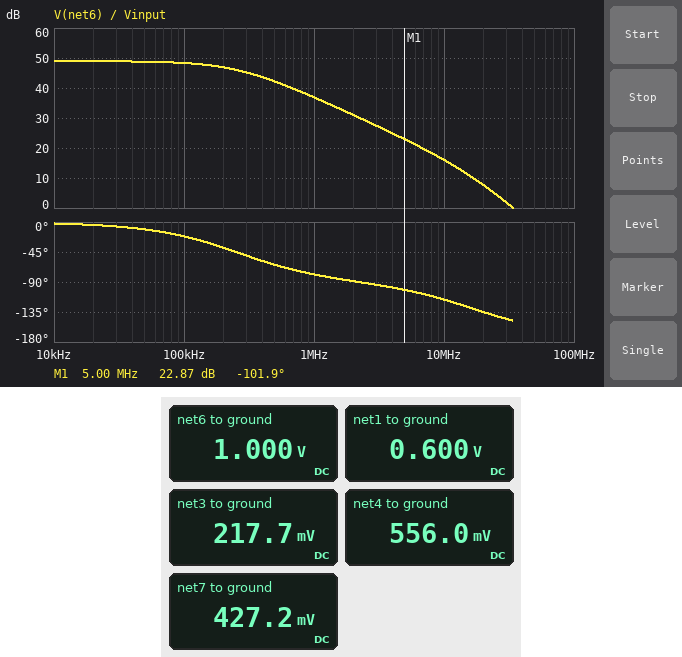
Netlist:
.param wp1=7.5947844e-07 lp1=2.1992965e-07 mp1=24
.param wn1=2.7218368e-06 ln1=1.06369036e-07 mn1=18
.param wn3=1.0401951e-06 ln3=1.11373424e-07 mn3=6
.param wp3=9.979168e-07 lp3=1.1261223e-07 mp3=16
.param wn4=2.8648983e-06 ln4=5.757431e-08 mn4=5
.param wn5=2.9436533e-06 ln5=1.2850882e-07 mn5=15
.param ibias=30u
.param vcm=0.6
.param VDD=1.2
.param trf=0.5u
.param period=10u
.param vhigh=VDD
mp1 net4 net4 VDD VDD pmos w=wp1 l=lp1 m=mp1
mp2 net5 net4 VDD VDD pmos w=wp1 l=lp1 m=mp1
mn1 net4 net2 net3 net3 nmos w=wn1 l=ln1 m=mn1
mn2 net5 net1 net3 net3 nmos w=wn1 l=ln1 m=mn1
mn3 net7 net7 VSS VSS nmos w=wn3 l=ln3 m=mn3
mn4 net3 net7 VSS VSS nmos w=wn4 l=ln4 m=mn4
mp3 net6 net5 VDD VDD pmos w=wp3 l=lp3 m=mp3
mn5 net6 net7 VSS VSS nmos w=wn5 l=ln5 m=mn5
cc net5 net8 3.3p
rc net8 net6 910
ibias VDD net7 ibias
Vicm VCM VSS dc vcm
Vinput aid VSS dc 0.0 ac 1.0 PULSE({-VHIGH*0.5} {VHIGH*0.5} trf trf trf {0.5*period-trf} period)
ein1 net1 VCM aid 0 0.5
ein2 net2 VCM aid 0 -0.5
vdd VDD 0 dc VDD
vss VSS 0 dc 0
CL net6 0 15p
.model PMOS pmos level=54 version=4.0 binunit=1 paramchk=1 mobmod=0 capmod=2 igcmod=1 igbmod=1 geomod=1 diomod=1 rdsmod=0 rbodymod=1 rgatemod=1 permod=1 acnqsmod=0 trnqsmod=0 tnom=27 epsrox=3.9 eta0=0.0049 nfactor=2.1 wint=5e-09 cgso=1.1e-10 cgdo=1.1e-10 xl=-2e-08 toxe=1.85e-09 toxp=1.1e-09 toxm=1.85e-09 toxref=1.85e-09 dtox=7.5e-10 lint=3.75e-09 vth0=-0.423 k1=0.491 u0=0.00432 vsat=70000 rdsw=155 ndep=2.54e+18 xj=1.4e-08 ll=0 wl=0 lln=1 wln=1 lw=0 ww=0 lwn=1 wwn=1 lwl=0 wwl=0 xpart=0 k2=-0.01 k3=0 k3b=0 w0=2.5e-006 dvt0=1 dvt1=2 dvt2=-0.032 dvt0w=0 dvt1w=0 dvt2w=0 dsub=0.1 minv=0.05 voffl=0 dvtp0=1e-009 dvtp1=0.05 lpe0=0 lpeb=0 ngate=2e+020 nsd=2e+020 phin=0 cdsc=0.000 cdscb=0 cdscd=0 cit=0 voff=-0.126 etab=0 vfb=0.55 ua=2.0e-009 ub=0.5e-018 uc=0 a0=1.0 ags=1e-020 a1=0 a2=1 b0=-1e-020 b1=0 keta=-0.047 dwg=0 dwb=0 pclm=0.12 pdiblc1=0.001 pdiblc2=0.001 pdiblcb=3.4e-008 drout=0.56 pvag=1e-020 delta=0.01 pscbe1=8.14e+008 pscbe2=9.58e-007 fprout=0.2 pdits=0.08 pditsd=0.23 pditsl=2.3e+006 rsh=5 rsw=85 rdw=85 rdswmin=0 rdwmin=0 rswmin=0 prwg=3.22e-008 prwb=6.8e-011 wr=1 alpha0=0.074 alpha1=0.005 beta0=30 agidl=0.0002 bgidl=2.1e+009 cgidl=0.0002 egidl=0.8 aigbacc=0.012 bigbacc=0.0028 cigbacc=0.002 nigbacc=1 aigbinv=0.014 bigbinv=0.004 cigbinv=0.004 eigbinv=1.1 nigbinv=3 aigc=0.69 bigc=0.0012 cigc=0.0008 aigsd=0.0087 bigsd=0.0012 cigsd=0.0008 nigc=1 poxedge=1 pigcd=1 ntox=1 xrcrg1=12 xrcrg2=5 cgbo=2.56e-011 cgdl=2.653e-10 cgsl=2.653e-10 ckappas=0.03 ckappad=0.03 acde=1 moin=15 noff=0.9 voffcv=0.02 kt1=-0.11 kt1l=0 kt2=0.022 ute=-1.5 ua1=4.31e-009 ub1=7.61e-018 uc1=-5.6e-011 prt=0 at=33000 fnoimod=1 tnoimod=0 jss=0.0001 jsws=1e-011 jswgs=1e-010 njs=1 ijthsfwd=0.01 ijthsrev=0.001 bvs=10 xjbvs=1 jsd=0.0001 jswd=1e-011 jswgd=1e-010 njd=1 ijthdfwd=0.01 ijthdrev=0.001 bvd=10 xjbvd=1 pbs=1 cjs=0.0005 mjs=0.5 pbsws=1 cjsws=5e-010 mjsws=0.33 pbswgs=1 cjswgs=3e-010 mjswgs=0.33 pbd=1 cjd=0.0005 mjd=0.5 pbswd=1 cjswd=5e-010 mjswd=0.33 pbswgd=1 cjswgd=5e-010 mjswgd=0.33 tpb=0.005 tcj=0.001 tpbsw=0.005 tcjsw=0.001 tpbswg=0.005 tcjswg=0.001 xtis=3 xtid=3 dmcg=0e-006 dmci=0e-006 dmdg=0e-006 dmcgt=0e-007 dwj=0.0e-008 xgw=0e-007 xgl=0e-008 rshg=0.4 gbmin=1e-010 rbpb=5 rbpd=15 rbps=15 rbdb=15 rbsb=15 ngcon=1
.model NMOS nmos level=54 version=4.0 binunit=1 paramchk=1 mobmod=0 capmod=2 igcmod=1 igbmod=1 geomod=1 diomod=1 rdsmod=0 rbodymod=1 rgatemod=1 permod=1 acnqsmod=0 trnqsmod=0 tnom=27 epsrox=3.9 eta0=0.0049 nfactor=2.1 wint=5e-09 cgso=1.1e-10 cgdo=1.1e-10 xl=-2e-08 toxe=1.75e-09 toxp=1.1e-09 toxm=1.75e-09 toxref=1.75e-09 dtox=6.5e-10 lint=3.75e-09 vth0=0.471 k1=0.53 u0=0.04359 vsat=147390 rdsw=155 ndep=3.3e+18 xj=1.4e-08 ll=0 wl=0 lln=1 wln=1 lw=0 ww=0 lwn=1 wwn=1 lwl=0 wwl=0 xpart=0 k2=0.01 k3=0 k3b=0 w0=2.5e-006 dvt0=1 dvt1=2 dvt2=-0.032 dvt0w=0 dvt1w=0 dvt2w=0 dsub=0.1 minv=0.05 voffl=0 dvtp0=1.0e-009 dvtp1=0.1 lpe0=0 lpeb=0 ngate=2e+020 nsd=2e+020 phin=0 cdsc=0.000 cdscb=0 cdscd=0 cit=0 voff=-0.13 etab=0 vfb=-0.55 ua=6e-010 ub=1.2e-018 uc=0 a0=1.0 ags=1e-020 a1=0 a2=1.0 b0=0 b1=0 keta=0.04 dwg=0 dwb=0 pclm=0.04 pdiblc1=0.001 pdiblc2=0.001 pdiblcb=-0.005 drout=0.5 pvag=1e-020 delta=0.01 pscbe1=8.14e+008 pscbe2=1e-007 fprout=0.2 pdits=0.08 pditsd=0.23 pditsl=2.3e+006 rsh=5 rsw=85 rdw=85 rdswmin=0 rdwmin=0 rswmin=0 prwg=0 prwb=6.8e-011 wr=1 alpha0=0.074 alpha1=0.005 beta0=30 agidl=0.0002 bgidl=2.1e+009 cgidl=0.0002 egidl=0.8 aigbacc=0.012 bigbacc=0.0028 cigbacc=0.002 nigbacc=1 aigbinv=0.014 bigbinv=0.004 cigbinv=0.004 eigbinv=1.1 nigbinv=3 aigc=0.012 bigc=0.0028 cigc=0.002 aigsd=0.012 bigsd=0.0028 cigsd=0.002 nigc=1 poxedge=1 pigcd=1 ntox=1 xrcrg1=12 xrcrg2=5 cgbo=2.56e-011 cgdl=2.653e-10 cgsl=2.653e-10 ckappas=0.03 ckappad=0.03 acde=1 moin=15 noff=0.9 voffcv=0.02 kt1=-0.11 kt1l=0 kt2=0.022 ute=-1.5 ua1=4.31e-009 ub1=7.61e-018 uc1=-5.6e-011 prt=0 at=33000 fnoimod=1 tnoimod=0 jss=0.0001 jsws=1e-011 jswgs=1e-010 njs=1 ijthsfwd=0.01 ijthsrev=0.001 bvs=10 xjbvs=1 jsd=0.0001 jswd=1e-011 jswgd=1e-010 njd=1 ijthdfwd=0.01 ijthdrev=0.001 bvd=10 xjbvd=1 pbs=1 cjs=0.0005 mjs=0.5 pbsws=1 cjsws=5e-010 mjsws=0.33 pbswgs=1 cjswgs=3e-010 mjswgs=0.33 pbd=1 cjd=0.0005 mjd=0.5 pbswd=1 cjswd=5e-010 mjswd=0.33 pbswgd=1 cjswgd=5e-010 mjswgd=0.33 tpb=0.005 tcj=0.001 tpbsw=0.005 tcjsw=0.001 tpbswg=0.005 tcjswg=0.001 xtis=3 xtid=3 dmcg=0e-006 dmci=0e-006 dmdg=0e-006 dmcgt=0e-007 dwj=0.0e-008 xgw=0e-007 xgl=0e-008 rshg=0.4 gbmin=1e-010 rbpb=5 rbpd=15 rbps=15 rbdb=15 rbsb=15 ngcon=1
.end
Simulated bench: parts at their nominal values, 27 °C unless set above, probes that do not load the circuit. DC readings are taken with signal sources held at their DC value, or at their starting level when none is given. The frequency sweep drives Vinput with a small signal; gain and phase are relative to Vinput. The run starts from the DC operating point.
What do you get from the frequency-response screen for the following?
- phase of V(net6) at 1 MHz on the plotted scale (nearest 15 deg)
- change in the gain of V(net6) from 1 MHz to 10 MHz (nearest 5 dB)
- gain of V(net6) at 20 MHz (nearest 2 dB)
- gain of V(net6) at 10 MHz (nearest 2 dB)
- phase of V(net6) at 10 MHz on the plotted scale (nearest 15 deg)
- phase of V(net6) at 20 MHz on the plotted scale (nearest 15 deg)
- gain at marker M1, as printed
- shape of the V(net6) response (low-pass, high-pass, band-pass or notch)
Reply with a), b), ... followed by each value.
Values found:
a) -75 deg
b) -20 dB
c) 8 dB
d) 16 dB
e) -120 deg
f) -135 deg
g) 22.87 dB
h) low-pass
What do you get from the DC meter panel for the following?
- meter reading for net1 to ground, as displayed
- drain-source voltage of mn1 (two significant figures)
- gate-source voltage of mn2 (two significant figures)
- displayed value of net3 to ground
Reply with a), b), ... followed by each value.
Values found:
a) 0.600 V
b) 340 mV
c) 380 mV
d) 217.7 mV
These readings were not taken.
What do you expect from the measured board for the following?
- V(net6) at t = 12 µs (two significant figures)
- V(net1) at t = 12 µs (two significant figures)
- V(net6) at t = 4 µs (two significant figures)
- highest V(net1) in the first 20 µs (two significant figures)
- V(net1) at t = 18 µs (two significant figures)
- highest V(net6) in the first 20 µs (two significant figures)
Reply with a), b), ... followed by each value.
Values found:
a) 1.2 V
b) 900 mV
c) 1.2 V
d) 900 mV
e) 300 mV
f) 1.2 V
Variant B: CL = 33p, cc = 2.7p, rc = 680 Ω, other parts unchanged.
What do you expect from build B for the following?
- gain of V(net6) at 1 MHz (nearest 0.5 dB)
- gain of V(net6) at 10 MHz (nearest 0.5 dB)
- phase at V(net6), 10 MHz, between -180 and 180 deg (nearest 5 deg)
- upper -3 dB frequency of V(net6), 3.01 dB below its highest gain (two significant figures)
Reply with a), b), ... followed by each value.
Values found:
a) 37.5 dB
b) 14.5 dB
c) -135 deg
d) 280 kHz
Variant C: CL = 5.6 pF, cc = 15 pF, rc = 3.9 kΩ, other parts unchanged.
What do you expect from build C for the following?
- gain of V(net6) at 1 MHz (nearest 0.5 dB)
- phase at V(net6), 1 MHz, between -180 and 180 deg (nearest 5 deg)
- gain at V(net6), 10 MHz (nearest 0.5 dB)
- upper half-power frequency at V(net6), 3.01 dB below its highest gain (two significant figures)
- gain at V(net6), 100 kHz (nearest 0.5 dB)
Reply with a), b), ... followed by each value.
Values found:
a) 25.0 dB
b) -70 deg
c) 14.0 dB
d) 60 kHz
e) 43.0 dB
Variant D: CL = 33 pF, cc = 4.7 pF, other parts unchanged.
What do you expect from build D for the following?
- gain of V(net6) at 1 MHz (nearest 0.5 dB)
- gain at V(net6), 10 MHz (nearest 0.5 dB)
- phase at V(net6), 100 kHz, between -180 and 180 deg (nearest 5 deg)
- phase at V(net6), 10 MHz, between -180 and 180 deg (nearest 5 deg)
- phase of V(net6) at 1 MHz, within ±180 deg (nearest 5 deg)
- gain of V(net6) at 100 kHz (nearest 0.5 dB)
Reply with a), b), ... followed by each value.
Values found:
a) 33.5 dB
b) 10.0 dB
c) -30 deg
d) -135 deg
e) -85 deg
f) 47.5 dB
